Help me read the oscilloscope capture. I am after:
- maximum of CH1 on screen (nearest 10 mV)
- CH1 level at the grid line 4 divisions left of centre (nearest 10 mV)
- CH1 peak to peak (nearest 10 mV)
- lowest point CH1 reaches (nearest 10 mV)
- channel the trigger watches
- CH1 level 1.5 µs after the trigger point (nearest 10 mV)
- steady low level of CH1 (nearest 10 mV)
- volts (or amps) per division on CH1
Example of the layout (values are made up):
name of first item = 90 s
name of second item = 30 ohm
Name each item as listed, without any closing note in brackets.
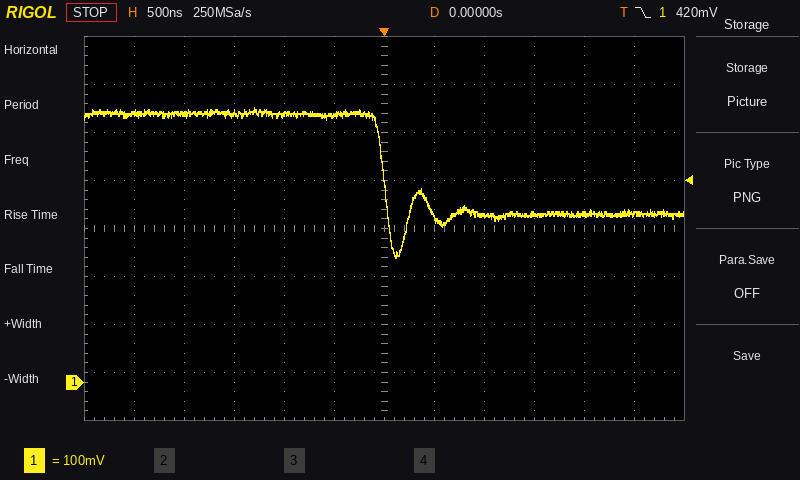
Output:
maximum of CH1 on screen = 570 mV
CH1 level at the grid line 4 divisions left of centre = 560 mV
CH1 peak to peak = 310 mV
lowest point CH1 reaches = 260 mV
channel the trigger watches = CH1
CH1 level 1.5 µs after the trigger point = 350 mV
steady low level of CH1 = 350 mV
volts (or amps) per division on CH1 = 100 mV
